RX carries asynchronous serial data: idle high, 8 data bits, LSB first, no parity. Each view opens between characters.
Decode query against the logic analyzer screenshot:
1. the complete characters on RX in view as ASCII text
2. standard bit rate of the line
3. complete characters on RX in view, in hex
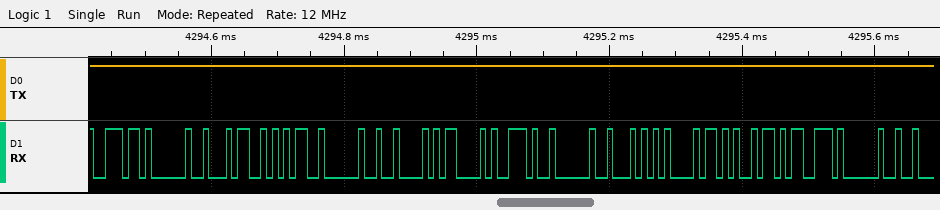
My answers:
"n 45 BC. This "
115200 baud
6E, 20, 34, 35, 20, 42, 43, 2E, 20, 54, 68, 69, 73, 20
